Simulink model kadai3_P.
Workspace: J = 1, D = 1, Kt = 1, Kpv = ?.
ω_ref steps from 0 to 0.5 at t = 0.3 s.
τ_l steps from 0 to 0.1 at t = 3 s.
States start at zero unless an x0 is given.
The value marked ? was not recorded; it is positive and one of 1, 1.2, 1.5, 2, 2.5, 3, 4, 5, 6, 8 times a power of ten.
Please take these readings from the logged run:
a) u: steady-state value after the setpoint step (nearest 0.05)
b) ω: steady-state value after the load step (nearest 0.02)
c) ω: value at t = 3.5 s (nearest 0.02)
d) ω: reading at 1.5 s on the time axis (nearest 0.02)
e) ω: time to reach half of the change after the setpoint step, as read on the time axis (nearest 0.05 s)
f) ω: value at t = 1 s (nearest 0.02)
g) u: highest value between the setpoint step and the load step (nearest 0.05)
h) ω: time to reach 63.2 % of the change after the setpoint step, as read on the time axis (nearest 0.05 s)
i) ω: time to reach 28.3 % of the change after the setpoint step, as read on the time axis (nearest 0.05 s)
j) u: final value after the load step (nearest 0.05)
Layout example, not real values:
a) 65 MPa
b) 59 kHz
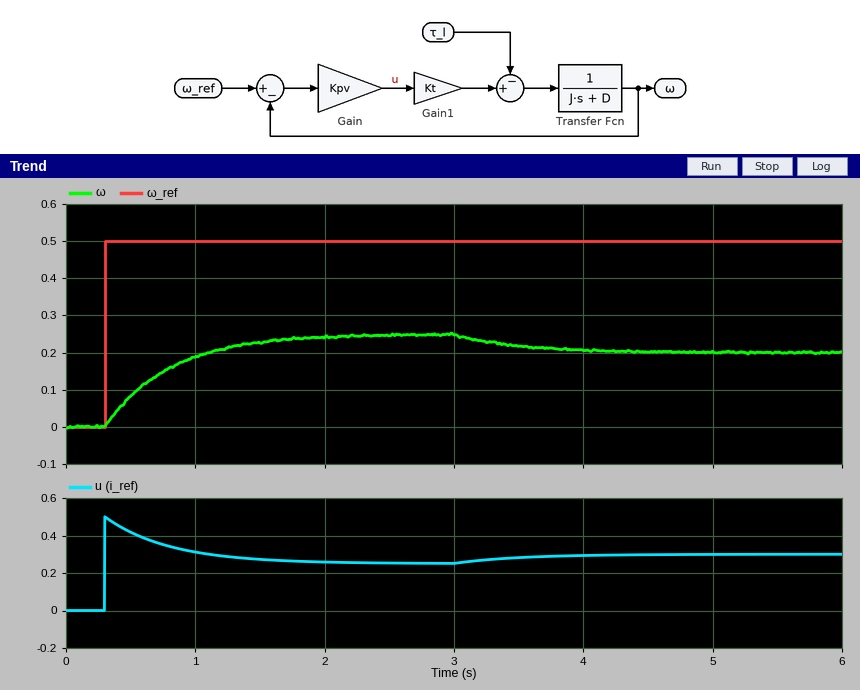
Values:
a) 0.25
b) 0.20
c) 0.22
d) 0.22
e) 0.65 s
f) 0.18
g) 0.50
h) 0.80 s
i) 0.45 s
j) 0.30
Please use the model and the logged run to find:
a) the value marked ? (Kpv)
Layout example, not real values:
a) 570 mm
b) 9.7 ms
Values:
a) 1
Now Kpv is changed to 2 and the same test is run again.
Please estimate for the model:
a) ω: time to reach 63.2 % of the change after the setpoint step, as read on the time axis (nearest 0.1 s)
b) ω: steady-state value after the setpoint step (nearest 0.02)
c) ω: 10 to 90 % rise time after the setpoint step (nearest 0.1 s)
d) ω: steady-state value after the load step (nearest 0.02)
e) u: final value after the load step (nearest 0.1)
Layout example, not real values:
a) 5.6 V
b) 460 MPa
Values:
a) 0.6 s
b) 0.34
c) 0.7 s
d) 0.30
e) 0.4
